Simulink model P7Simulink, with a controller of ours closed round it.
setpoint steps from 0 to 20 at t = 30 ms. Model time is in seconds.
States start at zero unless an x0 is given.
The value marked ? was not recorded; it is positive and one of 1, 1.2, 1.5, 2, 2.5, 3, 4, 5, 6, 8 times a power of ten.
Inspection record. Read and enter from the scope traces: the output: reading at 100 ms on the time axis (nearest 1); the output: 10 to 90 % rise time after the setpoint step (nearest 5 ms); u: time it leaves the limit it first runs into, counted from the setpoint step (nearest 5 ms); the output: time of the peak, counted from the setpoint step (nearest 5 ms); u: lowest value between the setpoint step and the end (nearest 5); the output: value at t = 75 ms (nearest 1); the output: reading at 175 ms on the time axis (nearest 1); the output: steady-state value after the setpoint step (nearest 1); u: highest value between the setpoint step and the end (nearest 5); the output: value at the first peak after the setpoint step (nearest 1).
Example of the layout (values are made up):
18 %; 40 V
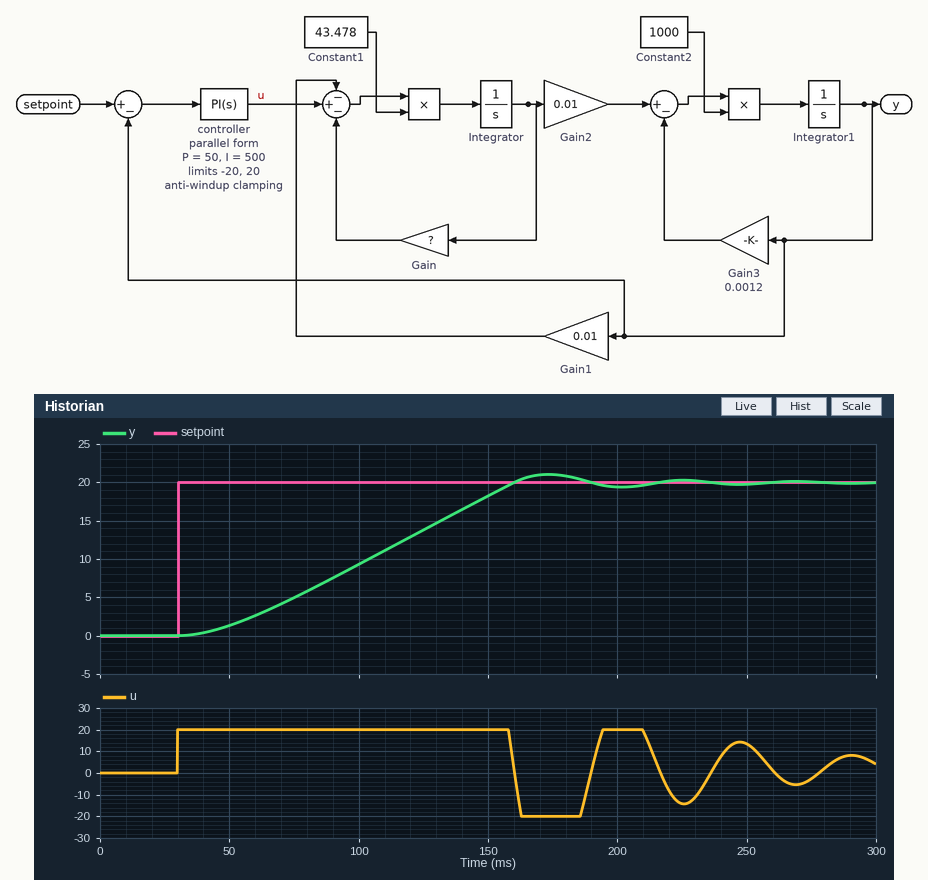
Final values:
9; 95 ms; 130 ms; 145 ms; -20; 5; 21; 20; 20; 21
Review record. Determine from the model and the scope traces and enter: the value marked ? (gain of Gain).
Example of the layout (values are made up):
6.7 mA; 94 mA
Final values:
1
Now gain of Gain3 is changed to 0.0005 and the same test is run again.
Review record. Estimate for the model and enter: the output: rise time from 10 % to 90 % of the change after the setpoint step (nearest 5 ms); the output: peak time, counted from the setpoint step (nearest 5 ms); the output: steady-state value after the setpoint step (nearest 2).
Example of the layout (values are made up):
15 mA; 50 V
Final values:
90 ms; 140 ms; 20
